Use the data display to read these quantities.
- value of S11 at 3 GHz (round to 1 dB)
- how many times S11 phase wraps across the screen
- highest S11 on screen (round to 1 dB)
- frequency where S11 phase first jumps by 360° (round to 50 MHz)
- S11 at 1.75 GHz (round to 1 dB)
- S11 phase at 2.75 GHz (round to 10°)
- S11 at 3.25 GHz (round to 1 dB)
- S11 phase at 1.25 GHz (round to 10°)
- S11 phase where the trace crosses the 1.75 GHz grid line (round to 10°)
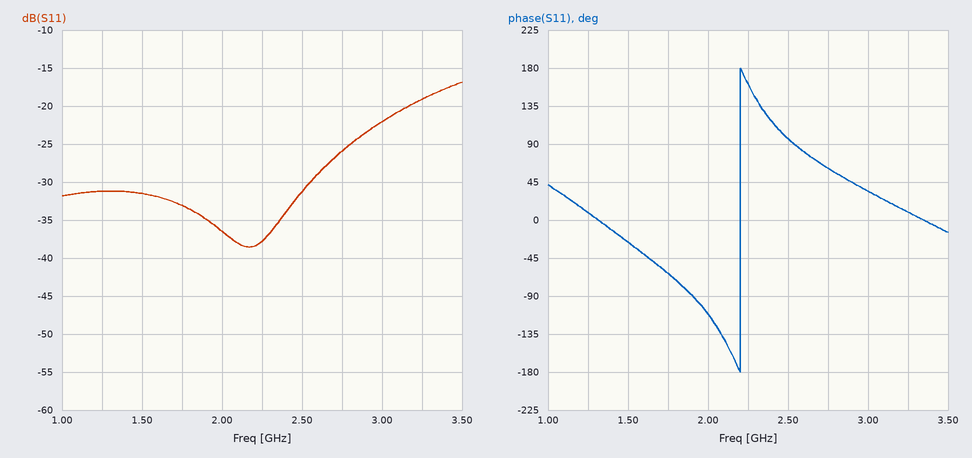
-22 dB
1
-17 dB
2.20 GHz
-33 dB
60°
-19 dB
10°
-60°
